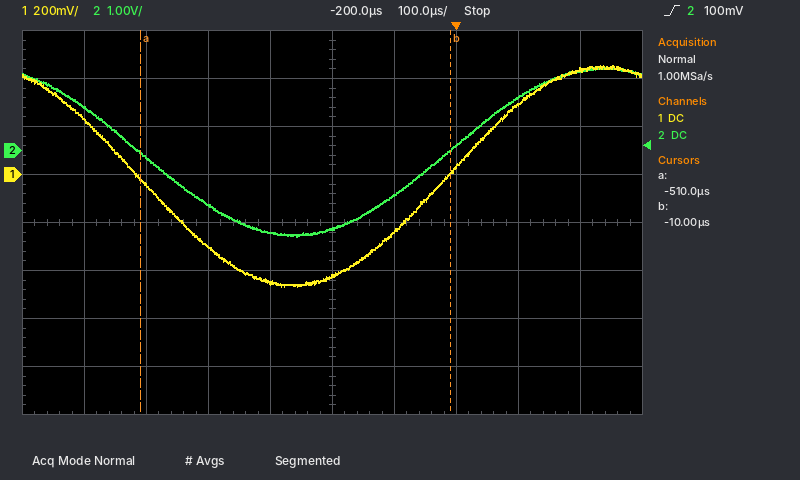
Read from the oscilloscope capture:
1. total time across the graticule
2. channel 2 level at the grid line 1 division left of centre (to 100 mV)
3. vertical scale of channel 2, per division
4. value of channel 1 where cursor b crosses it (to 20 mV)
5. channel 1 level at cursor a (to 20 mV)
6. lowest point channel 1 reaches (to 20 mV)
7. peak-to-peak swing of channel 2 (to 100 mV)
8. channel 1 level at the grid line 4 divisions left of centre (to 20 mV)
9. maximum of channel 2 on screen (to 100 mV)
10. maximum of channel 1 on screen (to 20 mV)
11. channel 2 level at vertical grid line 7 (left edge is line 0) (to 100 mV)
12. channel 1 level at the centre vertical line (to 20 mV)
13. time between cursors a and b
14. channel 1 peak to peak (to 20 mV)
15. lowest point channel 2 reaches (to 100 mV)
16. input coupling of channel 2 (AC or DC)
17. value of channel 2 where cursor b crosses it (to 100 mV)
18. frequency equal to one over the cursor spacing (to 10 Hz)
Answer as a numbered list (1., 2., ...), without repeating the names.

1. 1 ms
2. -1.7 V
3. 1 V
4. 0 mV
5. -20 mV
6. -460 mV
7. 3.5 V
8. 240 mV
9. 1.7 V
10. 460 mV
11. 100 mV
12. -420 mV
13. 500 µs
14. 920 mV
15. -1.8 V
16. DC
17. 0.0 V
18. 2.00 kHz
